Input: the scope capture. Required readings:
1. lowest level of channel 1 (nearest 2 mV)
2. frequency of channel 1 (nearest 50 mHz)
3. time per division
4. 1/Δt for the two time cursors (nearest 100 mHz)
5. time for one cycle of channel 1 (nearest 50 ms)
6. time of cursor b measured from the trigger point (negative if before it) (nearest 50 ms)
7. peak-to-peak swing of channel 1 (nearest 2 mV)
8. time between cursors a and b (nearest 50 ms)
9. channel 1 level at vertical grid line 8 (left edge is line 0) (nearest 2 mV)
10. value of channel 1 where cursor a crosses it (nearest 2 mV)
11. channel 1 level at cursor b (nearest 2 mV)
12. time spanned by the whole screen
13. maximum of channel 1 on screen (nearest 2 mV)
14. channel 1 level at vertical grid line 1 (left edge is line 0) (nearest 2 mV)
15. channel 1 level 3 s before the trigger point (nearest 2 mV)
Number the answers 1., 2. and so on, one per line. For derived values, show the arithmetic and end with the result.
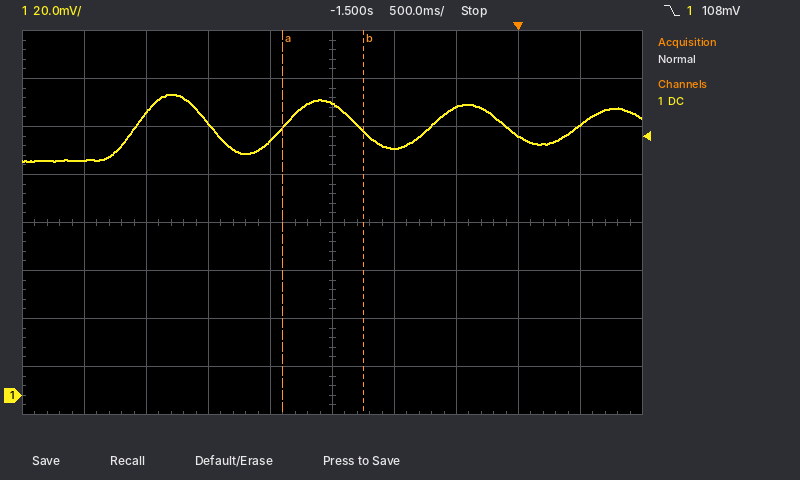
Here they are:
1. 98 mV
2. 1 / 1.20 s ≈ 833 mHz, so 850 mHz to the nearest 50 mHz
3. 500 ms
4. 1 / 650 ms ≈ 1.5 Hz
5. 1.20 s
6. -1.25 s
7. 126 mV − (98 mV) = 28 mV
8. 650 ms
9. 108 mV
10. 112 mV
11. 110 mV
12. 5 s
13. 126 mV
14. 98 mV
15. 118 mV
